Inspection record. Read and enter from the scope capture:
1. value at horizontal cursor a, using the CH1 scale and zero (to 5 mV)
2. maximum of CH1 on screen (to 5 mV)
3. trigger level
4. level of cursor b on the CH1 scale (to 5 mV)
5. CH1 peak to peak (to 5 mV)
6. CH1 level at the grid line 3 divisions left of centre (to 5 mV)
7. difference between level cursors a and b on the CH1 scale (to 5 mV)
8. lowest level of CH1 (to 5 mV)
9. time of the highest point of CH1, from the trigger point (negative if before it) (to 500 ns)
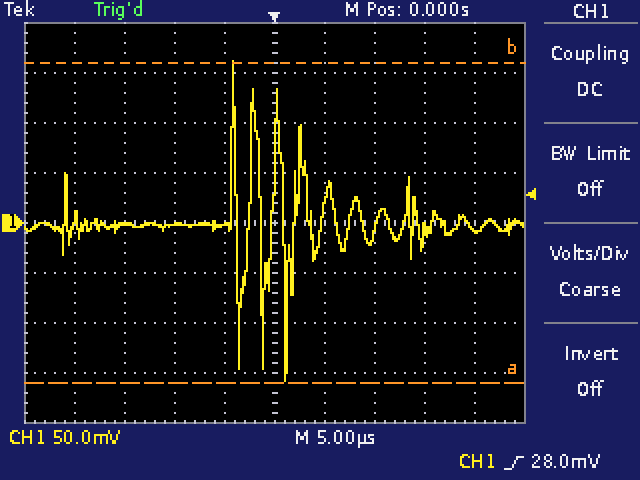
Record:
-160 mV
160 mV
28.0 mV
160 mV
320 mV
0 mV
320 mV
-160 mV
-4.0 µs
